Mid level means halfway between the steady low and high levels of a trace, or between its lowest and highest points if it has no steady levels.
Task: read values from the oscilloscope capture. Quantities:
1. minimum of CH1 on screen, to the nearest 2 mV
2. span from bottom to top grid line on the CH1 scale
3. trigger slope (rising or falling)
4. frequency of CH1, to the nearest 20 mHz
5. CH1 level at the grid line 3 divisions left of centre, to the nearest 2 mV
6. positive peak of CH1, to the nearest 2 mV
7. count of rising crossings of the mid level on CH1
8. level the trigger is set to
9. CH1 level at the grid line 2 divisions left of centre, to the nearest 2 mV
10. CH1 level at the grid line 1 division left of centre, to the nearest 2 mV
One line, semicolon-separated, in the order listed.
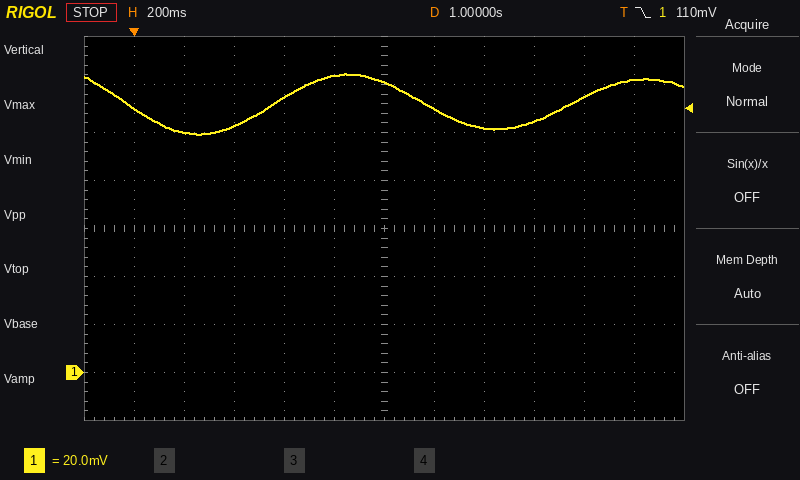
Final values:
100 mV; 160 mV; falling; 840 mHz; 102 mV; 124 mV; 2; 110 mV; 114 mV; 124 mV
